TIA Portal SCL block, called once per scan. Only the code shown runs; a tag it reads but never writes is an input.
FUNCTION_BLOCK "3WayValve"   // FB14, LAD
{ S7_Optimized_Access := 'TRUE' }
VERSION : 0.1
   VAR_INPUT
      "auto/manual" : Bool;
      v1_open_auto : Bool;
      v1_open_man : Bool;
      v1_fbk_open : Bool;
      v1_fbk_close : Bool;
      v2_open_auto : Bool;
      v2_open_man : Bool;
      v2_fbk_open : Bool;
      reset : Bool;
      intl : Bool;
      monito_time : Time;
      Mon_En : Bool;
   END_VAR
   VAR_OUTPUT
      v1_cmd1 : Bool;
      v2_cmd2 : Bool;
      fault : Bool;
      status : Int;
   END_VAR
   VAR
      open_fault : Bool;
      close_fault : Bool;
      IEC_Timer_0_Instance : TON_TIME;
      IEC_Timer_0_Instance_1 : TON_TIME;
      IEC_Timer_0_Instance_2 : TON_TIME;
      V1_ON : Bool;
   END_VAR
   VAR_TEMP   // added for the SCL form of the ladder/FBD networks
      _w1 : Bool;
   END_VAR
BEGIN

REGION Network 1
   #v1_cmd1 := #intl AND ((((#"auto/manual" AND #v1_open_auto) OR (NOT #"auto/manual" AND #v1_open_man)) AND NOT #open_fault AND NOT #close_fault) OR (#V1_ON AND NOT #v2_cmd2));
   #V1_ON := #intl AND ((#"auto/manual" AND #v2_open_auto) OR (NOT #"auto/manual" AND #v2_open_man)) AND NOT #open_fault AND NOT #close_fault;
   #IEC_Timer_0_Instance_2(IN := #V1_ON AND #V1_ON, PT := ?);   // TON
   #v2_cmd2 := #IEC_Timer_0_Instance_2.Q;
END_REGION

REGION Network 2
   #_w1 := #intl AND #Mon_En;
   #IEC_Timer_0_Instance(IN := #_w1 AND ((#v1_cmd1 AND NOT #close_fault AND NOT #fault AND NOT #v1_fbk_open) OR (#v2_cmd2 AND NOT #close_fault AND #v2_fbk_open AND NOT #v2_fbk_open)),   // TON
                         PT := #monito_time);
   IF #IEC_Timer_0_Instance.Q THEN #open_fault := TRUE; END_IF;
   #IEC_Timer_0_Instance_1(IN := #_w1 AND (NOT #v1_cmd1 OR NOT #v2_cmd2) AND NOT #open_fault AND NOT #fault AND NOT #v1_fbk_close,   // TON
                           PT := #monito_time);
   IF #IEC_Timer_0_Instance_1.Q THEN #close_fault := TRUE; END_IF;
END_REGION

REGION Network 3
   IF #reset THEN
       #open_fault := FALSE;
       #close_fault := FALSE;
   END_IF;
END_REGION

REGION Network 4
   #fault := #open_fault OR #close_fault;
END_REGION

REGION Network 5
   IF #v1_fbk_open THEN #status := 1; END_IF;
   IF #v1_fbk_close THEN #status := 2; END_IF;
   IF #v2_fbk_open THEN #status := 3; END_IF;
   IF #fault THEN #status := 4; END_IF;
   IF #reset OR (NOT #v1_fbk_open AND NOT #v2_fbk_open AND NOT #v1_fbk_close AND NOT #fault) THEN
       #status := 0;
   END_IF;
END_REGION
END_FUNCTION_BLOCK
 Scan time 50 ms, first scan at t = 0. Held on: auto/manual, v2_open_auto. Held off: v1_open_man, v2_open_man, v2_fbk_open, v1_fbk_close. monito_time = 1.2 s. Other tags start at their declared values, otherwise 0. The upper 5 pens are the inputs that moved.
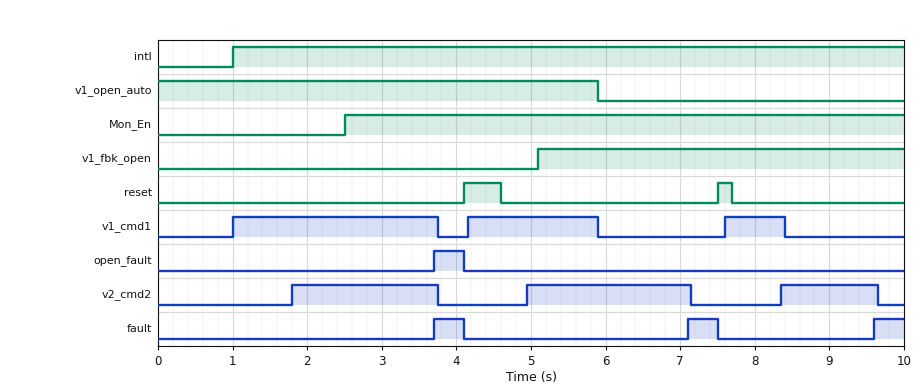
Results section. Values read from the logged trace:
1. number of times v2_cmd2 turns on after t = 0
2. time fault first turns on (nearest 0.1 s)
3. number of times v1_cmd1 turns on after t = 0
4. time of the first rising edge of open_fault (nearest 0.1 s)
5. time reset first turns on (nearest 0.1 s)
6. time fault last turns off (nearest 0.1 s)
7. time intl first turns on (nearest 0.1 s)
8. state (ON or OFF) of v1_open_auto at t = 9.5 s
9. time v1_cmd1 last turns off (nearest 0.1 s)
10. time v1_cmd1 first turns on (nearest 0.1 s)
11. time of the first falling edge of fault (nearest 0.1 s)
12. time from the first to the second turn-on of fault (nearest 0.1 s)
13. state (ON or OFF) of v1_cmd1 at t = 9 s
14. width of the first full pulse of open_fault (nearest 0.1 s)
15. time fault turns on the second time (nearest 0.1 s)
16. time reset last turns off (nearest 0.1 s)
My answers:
3
3.7 s
3
3.7 s
4.1 s
7.5 s
1.0 s
OFF
8.4 s
1.0 s
4.1 s
3.4 s
OFF
0.4 s
7.1 s
7.7 s
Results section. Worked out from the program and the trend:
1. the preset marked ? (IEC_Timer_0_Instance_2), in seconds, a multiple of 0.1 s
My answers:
0.8 s
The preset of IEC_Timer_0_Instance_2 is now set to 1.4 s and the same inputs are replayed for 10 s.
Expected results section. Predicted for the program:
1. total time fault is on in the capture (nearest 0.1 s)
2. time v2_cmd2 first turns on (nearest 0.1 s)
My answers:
3.8 s
2.4 s
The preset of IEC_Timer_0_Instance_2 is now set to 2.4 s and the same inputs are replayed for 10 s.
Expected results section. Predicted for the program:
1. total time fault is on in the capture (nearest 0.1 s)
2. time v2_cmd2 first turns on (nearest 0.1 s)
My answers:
3.8 s
3.4 s
